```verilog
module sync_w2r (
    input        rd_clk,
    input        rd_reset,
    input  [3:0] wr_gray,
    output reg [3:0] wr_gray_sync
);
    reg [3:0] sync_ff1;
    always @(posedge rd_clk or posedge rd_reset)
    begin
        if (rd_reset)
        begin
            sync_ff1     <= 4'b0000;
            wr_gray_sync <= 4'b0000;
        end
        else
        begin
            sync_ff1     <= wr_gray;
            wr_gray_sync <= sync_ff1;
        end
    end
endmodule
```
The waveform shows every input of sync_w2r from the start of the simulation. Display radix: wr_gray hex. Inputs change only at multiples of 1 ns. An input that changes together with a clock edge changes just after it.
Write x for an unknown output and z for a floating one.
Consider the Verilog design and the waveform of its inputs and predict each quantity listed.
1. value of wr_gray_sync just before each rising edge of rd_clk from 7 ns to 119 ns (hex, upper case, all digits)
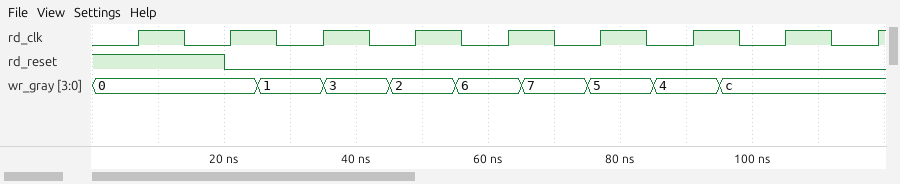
0, 0, 0, 0, 1, 2, 6, 5, 4
